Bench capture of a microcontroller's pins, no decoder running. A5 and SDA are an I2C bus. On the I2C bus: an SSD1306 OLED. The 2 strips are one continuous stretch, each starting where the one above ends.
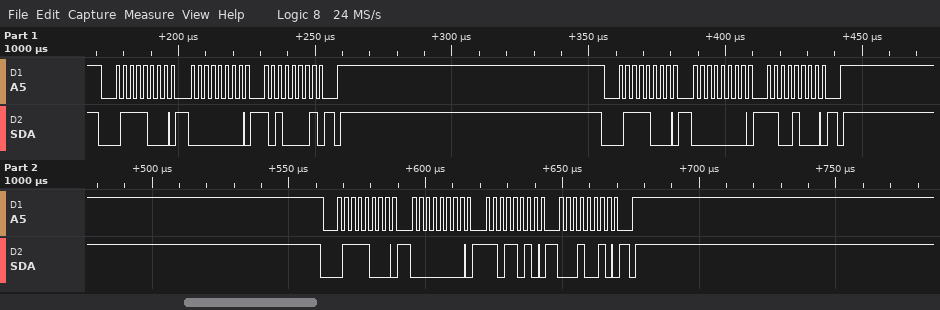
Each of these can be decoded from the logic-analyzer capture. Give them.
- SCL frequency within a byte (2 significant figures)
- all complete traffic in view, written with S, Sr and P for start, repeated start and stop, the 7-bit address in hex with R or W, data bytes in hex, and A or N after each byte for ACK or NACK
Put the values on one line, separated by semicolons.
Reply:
400 kHz; S 3CW A 00 A A1 A P S 3CW A 00 A C8 A P S 3CW A 00 A DA A 12 A P
